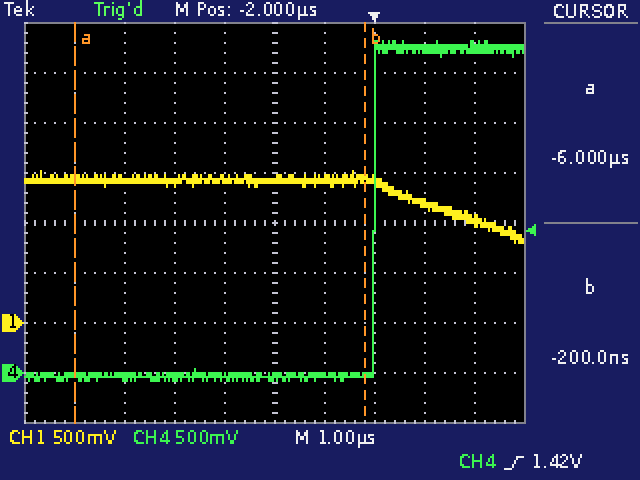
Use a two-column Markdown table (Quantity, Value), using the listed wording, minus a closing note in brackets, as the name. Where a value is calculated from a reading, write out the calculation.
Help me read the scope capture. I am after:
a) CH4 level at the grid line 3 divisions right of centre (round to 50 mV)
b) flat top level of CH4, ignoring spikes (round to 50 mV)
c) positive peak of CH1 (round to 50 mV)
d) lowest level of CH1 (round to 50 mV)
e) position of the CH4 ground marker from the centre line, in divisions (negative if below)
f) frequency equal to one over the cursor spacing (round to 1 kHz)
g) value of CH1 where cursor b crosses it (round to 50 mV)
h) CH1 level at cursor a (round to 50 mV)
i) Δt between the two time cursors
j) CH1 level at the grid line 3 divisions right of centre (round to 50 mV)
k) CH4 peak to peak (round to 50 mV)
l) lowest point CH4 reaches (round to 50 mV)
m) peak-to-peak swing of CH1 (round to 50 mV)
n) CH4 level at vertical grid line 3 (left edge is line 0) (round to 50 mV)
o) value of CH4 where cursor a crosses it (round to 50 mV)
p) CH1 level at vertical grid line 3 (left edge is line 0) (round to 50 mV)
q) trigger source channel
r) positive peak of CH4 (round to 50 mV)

| Quantity | Value |
|---|---|
| CH4 level at the grid line 3 divisions right of centre | 3.25 V |
| flat top level of CH4, ignoring spikes | 3.25 V |
| positive peak of CH1 | 1.50 V |
| lowest level of CH1 | 800 mV |
| position of the CH4 ground marker from the centre line, in divisions | -3.0 div |
| frequency equal to one over the cursor spacing | 1 / 5.8 µs ≈ 172 kHz |
| value of CH1 where cursor b crosses it | 1.45 V |
| CH1 level at cursor a | 1.45 V |
| Δt between the two time cursors | -200 ns − (-6 µs) = 5.8 µs |
| CH1 level at the grid line 3 divisions right of centre | 1.20 V |
| CH4 peak to peak | 3.30 V − (-100 mV) = 3.40 V |
| lowest point CH4 reaches | -100 mV |
| peak-to-peak swing of CH1 | 1.50 V − (800 mV) = 700 mV |
| CH4 level at vertical grid line 3 (left edge is line 0) | -50 mV |
| value of CH4 where cursor a crosses it | -50 mV |
| CH1 level at vertical grid line 3 (left edge is line 0) | 1.40 V |
| trigger source channel | CH4 |
| positive peak of CH4 | 3.30 V |
